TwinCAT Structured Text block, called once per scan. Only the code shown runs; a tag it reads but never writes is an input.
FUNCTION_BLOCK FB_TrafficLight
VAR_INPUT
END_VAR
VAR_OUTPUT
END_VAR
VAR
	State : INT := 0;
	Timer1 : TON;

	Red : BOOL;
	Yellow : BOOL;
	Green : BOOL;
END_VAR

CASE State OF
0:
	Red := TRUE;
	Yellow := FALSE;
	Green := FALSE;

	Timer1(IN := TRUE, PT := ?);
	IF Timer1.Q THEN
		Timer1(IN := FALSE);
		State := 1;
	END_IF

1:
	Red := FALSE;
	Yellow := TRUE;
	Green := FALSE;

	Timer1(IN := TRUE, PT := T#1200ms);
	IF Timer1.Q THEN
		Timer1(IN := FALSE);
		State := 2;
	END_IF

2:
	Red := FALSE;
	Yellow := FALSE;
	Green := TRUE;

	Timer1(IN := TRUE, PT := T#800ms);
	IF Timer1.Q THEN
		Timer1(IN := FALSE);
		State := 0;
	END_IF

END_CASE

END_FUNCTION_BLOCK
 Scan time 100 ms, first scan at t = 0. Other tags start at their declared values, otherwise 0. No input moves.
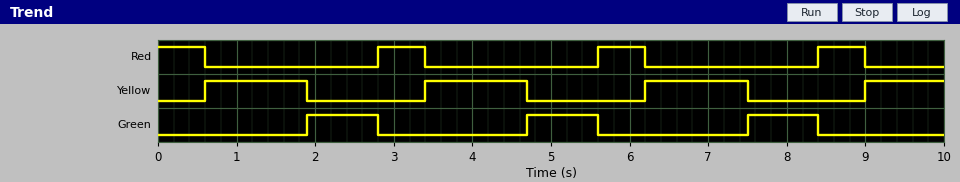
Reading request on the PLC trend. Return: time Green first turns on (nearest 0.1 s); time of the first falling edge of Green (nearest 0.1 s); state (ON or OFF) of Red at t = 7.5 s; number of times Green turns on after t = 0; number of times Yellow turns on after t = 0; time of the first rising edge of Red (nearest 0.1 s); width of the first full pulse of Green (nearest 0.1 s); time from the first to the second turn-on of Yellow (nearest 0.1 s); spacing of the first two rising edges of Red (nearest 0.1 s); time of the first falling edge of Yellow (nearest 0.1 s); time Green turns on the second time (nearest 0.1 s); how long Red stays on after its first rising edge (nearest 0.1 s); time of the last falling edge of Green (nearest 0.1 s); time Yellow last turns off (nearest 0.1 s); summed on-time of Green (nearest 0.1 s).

1.9 s
2.8 s
OFF
3
4
2.8 s
0.9 s
2.8 s
2.8 s
1.9 s
4.7 s
0.6 s
8.4 s
7.5 s
2.7 s
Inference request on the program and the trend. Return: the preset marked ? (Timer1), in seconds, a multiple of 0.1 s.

0.5 s
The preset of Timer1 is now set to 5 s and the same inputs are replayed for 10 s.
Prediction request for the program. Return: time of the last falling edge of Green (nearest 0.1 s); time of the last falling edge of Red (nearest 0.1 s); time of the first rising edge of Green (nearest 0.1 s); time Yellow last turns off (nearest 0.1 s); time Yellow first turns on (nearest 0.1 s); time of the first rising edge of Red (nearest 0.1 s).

7.3 s
5.1 s
6.4 s
6.4 s
5.1 s
7.3 s
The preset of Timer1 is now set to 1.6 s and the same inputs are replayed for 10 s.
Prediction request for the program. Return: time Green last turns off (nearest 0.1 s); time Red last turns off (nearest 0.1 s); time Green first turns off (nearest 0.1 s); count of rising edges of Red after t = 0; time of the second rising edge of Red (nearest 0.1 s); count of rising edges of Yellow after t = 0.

7.8 s
9.5 s
3.9 s
2
7.8 s
3
